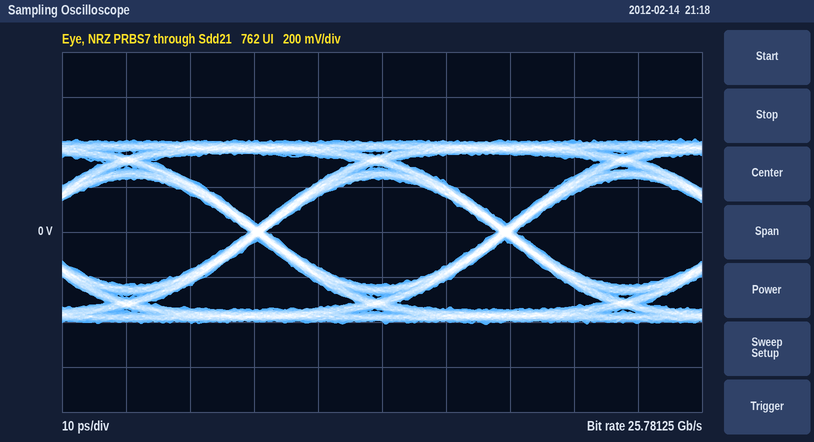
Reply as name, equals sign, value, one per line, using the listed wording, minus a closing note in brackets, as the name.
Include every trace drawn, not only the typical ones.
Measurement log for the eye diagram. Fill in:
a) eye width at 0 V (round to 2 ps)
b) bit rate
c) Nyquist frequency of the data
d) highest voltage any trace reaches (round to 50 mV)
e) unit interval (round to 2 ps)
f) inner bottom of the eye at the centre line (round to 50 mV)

eye width at 0 V = 36 ps
bit rate = 25.78125 Gb/s
Nyquist frequency of the data = 12.89062 GHz
highest voltage any trace reaches = 400 mV
unit interval = 38 ps
inner bottom of the eye at the centre line = -250 mV
